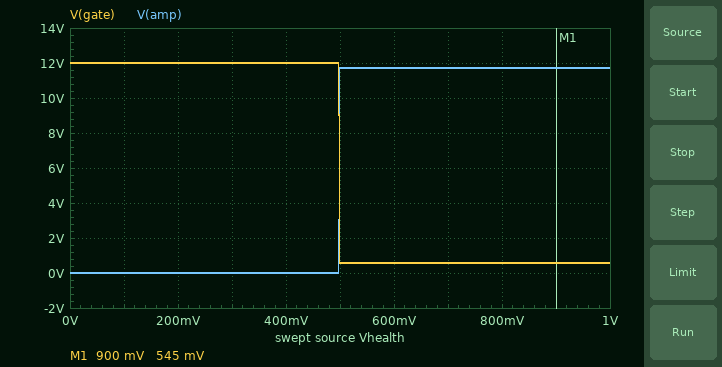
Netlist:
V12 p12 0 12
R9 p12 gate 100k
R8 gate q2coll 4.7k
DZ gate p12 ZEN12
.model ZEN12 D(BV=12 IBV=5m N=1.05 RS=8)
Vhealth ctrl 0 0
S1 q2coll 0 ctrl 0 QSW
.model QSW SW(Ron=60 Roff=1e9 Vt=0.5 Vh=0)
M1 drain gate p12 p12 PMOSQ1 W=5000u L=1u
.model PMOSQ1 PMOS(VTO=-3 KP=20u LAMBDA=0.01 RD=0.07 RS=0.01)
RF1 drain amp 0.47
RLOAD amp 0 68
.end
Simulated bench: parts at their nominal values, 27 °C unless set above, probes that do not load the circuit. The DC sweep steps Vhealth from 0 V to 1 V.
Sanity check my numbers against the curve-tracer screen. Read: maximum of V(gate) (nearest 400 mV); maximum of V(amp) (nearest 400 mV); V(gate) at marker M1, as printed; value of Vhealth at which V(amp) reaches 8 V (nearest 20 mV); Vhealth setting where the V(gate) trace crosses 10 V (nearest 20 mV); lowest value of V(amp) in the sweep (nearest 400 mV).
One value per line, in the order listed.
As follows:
12.0 V
11.6 V
545 mV
500 mV
500 mV
0 V
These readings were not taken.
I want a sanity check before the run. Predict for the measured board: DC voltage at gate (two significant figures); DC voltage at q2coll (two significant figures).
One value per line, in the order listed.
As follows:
12 V
12 V
